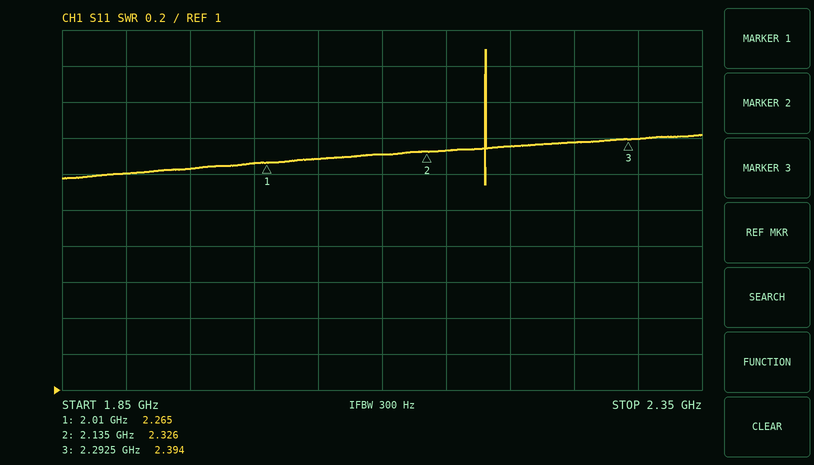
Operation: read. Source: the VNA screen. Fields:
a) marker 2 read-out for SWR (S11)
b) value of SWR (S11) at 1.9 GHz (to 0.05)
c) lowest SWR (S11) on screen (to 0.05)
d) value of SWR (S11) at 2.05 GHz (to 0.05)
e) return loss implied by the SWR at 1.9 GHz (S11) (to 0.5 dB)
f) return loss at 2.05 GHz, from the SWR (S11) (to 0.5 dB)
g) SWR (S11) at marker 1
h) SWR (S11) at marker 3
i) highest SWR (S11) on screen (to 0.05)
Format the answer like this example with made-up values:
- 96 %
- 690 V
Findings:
- 2.326
- 2.20
- 2.15
- 2.30
- 8.5 dB
- 8.0 dB
- 2.265
- 2.394
- 2.90
